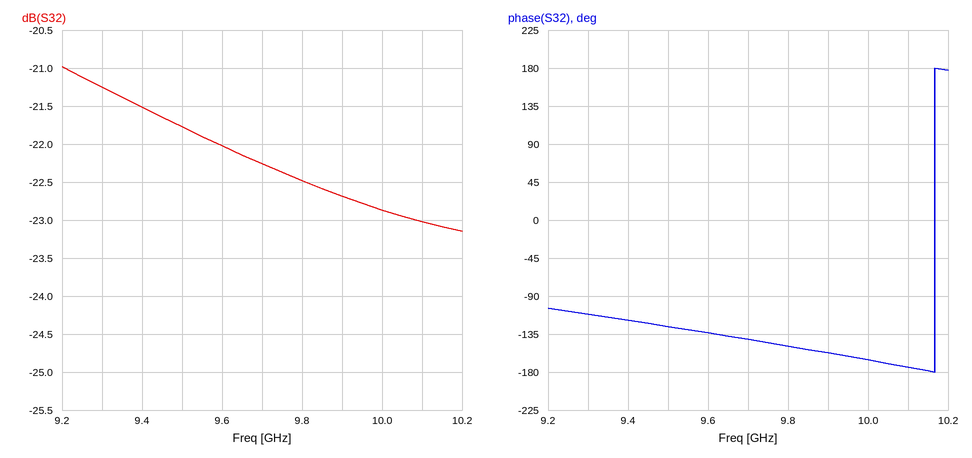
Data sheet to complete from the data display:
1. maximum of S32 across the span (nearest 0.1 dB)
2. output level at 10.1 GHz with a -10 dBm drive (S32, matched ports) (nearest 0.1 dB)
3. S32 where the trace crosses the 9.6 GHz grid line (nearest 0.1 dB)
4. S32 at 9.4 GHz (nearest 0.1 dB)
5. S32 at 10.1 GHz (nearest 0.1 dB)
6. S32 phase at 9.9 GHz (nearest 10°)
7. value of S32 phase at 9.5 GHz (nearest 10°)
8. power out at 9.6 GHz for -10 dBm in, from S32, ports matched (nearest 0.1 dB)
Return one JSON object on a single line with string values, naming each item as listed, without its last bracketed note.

{"maximum of S32 across the span": "-21.0 dB", "output level at 10.1 GHz with a -10 dBm drive (S32, matched ports)": "-33.0 dBm", "S32 where the trace crosses the 9.6 GHz grid line": "-22.0 dB", "S32 at 9.4 GHz": "-21.5 dB", "S32 at 10.1 GHz": "-23.0 dB", "S32 phase at 9.9 GHz": "-160°", "value of S32 phase at 9.5 GHz": "-130°", "power out at 9.6 GHz for -10 dBm in, from S32, ports matched": "-32.0 dBm"}
